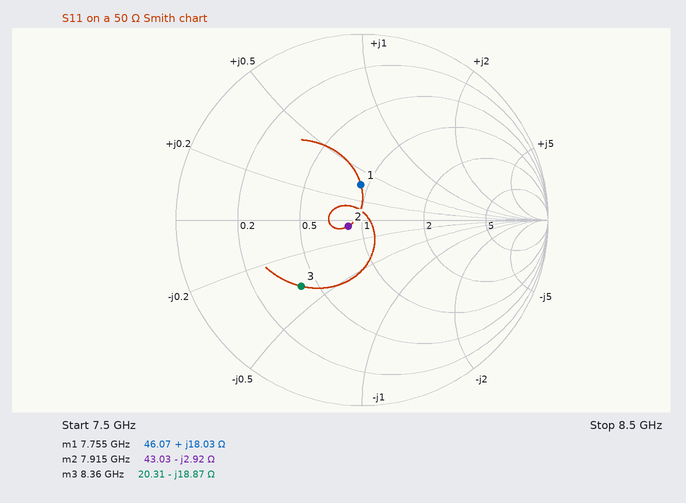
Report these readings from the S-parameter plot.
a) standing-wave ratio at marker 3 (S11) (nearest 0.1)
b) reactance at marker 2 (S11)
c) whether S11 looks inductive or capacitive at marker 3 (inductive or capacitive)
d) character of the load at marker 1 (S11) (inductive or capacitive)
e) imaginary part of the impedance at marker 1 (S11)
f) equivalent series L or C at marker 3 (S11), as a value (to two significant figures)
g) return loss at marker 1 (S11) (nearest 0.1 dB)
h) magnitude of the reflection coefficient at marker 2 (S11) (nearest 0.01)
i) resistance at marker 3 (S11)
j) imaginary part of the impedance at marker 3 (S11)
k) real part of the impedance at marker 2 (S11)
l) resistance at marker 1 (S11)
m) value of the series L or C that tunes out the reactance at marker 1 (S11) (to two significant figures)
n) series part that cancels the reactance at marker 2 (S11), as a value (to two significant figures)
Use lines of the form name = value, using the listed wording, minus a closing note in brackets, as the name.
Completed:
standing-wave ratio at marker 3 (S11) = 2.9
reactance at marker 2 = -2.92 Ω
whether S11 looks inductive or capacitive at marker 3 = capacitive
character of the load at marker 1 (S11) = inductive
imaginary part of the impedance at marker 1 = +18.03 Ω
equivalent series L or C at marker 3 (S11), as a value = 1.0 pF
return loss at marker 1 (S11) = 14.5 dB
magnitude of the reflection coefficient at marker 2 (S11) = 0.08
resistance at marker 3 = 20.31 Ω
imaginary part of the impedance at marker 3 = -18.87 Ω
real part of the impedance at marker 2 = 43.03 Ω
resistance at marker 1 = 46.07 Ω
value of the series L or C that tunes out the reactance at marker 1 (S11) = 1.1 pF
series part that cancels the reactance at marker 2 (S11), as a value = 59 pH
